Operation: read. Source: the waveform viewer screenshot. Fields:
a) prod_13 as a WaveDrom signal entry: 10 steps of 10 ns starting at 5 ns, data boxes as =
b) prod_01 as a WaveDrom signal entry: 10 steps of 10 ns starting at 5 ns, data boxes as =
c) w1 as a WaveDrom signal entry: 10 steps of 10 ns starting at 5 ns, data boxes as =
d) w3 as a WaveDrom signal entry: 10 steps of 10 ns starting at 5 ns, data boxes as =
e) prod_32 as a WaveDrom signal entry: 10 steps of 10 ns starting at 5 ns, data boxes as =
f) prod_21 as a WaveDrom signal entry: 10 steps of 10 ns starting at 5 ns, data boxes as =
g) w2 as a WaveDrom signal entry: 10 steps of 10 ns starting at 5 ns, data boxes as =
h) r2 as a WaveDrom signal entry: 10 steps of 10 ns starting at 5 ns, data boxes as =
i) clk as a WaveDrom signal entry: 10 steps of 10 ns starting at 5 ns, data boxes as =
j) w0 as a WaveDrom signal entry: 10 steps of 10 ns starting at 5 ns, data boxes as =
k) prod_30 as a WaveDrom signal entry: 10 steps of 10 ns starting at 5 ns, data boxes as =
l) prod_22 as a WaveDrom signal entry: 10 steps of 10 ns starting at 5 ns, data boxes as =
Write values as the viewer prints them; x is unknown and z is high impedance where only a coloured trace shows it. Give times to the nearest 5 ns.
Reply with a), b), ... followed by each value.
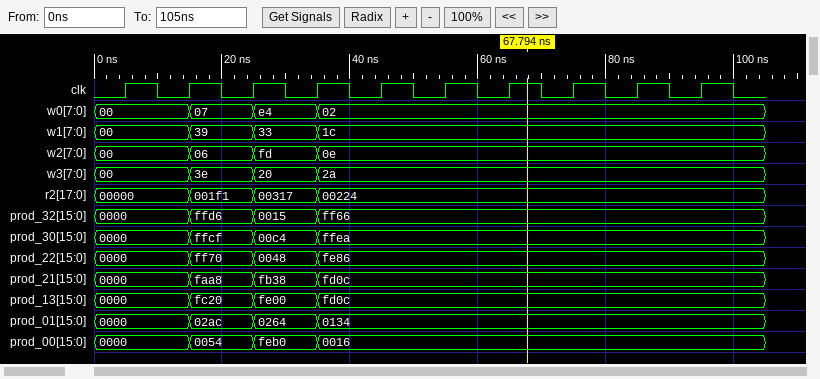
a) {name: 'prod_13', wave: '====......', data: '0000 fc20 fe00 fd0c'}
b) {name: 'prod_01', wave: '====......', data: '0000 02ac 0264 0134'}
c) {name: 'w1', wave: '====......', data: '00 39 33 1c'}
d) {name: 'w3', wave: '====......', data: '00 3e 20 2a'}
e) {name: 'prod_32', wave: '====......', data: '0000 ffd6 0015 ff66'}
f) {name: 'prod_21', wave: '====......', data: '0000 faa8 fb38 fd0c'}
g) {name: 'w2', wave: '====......', data: '00 06 fd 0e'}
h) {name: 'r2', wave: '====......', data: '00000 001f1 00317 00224'}
i) {name: 'clk', wave: 'p.........'}
j) {name: 'w0', wave: '====......', data: '00 07 e4 02'}
k) {name: 'prod_30', wave: '====......', data: '0000 ffcf 00c4 ffea'}
l) {name: 'prod_22', wave: '====......', data: '0000 ff70 0048 fe86'}
